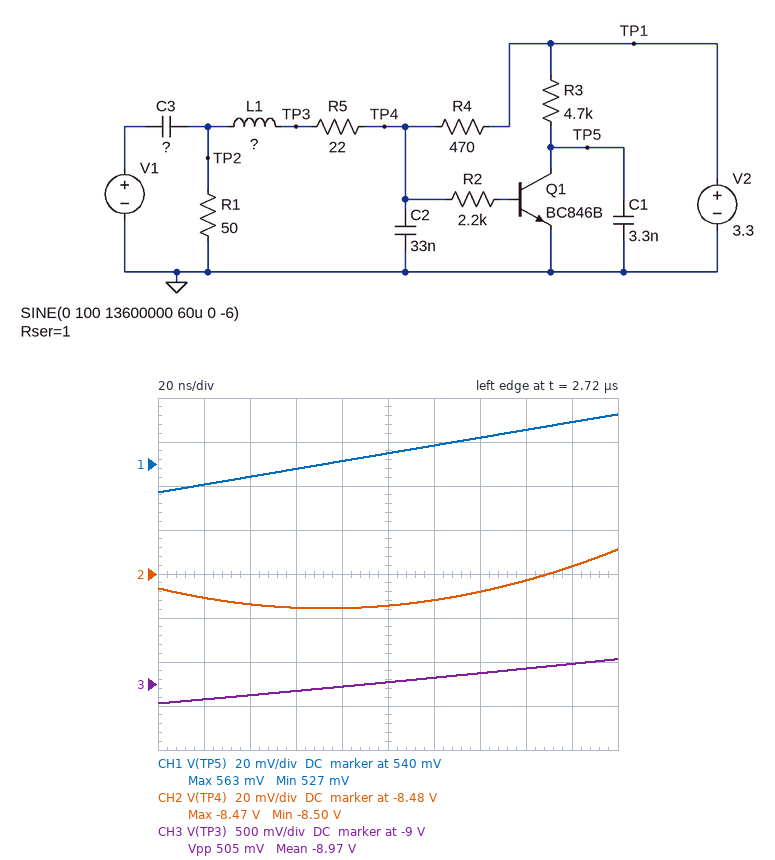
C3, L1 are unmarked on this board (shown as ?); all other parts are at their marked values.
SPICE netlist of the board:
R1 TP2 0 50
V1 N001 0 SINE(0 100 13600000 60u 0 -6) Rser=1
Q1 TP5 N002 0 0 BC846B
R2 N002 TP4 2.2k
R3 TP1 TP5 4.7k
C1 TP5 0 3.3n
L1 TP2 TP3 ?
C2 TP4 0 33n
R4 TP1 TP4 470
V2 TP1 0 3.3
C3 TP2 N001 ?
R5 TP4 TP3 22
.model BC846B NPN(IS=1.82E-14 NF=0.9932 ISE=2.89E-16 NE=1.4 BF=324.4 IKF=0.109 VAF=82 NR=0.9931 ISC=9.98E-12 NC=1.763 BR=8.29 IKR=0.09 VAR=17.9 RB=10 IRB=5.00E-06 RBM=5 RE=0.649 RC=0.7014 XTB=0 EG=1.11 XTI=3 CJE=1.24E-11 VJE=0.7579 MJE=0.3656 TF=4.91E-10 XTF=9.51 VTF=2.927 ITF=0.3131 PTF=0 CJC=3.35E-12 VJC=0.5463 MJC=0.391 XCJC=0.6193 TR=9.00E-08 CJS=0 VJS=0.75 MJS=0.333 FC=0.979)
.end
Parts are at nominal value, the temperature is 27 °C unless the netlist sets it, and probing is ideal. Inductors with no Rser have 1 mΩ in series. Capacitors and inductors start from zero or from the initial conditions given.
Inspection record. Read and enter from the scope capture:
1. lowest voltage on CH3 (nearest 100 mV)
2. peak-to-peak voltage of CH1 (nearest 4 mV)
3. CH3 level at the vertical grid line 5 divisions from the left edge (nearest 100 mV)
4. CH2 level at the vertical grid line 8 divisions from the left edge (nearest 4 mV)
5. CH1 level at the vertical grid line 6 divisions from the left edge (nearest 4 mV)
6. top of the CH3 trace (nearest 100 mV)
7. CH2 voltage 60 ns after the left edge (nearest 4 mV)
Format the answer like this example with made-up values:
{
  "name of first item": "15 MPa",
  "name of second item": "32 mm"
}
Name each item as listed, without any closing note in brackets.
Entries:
{
  "lowest voltage on CH3": "-9.2 V",
  "peak-to-peak voltage of CH1": "36 mV",
  "CH3 level at the vertical grid line 5 divisions from the left edge": "-9.0 V",
  "CH2 level at the vertical grid line 8 divisions from the left edge": "-8.484 V",
  "CH1 level at the vertical grid line 6 divisions from the left edge": "548 mV",
  "top of the CH3 trace": "-8.7 V",
  "CH2 voltage 60 ns after the left edge": "-8.496 V"
}
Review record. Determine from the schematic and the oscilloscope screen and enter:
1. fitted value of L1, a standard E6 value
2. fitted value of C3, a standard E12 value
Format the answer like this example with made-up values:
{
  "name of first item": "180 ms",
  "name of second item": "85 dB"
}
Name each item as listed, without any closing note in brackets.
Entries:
{
  "fitted value of L1, a standard E6 value": "33 µH",
  "fitted value of C3, a standard E12 value": "150 nF"
}
